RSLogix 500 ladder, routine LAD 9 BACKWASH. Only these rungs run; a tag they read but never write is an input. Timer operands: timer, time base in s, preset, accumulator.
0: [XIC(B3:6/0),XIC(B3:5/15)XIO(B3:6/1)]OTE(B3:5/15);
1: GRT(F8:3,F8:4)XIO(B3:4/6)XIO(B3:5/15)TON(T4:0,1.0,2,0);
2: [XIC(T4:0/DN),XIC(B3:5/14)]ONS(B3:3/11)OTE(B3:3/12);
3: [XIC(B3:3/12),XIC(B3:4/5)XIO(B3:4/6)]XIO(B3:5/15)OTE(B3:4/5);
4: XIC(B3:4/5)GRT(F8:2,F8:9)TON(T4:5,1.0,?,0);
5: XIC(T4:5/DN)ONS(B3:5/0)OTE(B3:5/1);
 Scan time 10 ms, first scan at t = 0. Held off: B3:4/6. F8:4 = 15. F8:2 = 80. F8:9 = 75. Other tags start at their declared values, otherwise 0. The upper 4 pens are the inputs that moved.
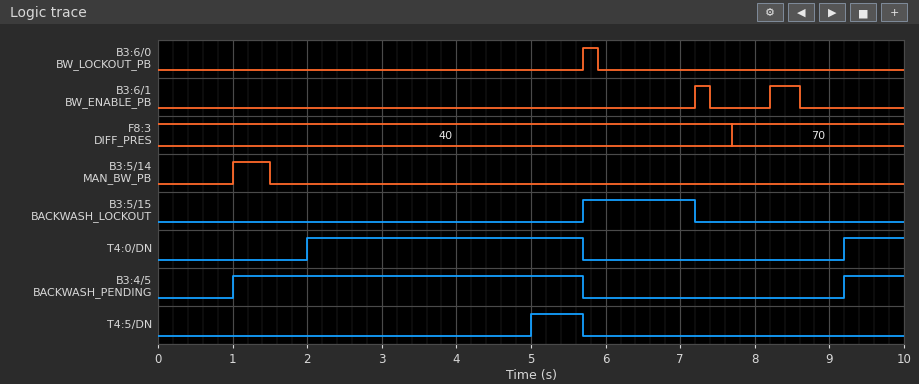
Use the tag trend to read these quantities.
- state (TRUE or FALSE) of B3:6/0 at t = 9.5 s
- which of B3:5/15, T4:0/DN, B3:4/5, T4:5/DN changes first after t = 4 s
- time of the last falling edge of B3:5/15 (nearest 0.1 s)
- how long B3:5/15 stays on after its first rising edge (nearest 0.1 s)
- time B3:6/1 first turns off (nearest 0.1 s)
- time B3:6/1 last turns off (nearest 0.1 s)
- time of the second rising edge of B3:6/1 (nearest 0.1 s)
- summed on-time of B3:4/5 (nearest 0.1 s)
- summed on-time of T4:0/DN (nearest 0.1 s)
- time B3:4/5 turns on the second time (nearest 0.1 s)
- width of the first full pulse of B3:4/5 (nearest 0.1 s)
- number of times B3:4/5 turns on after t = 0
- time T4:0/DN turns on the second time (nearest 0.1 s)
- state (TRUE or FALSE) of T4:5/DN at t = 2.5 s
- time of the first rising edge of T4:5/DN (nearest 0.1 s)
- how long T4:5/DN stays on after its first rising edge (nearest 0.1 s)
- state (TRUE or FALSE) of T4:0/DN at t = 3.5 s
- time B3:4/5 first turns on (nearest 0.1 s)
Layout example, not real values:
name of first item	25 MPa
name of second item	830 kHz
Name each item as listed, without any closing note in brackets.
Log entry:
state (TRUE or FALSE) of B3:6/0 at t = 9.5 s	FALSE
which of B3:5/15, T4:0/DN, B3:4/5, T4:5/DN changes first after t = 4 s	T4:5/DN
time of the last falling edge of B3:5/15	7.2 s
how long B3:5/15 stays on after its first rising edge	1.5 s
time B3:6/1 first turns off	7.4 s
time B3:6/1 last turns off	8.6 s
time of the second rising edge of B3:6/1	8.2 s
summed on-time of B3:4/5	5.5 s
summed on-time of T4:0/DN	4.5 s
time B3:4/5 turns on the second time	9.2 s
width of the first full pulse of B3:4/5	4.7 s
number of times B3:4/5 turns on after t = 0	2
time T4:0/DN turns on the second time	9.2 s
state (TRUE or FALSE) of T4:5/DN at t = 2.5 s	FALSE
time of the first rising edge of T4:5/DN	5.0 s
how long T4:5/DN stays on after its first rising edge	0.7 s
state (TRUE or FALSE) of T4:0/DN at t = 3.5 s	TRUE
time B3:4/5 first turns on	1.0 s
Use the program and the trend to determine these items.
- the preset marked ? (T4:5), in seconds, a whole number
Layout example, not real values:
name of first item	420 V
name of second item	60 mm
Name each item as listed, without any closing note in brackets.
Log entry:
the preset marked ? (T4:5), in seconds, a whole number	4 s
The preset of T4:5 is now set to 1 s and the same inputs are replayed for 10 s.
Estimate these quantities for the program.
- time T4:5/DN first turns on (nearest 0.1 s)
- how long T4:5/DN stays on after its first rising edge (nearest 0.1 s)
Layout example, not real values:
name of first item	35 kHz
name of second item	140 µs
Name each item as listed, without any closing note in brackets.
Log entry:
time T4:5/DN first turns on	2.0 s
how long T4:5/DN stays on after its first rising edge	3.7 s
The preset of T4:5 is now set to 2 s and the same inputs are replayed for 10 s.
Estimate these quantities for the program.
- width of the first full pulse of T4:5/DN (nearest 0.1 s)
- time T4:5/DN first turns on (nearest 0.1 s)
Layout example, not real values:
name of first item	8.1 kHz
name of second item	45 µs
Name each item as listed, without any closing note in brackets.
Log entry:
width of the first full pulse of T4:5/DN	2.7 s
time T4:5/DN first turns on	3.0 s
